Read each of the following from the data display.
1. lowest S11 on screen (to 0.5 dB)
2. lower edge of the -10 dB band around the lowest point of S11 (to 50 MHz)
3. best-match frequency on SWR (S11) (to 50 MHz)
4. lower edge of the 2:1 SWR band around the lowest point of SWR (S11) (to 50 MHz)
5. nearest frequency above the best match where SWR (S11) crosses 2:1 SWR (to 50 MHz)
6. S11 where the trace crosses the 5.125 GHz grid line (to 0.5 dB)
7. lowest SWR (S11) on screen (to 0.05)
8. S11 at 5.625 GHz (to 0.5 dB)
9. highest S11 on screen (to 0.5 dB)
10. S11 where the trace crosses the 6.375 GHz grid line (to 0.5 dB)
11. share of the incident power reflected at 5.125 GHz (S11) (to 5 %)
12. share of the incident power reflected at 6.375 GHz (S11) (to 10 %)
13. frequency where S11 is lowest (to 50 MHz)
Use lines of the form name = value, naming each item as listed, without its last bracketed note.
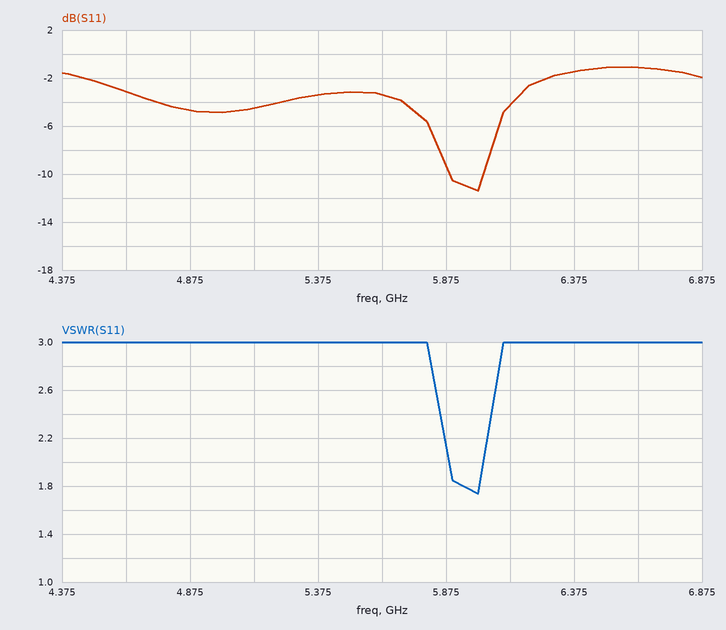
lowest S11 on screen = -11.5 dB
lower edge of the -10 dB band around the lowest point of S11 = 5.90 GHz
best-match frequency on SWR (S11) = 6.00 GHz
lower edge of the 2:1 SWR band around the lowest point of SWR (S11) = 5.90 GHz
nearest frequency above the best match where SWR (S11) crosses 2:1 SWR = 6.00 GHz
S11 where the trace crosses the 5.125 GHz grid line = -4.5 dB
lowest SWR (S11) on screen = 1.75
S11 at 5.625 GHz = -3.5 dB
highest S11 on screen = -1.0 dB
S11 where the trace crosses the 6.375 GHz grid line = -1.5 dB
share of the incident power reflected at 5.125 GHz (S11) = 35 %
share of the incident power reflected at 6.375 GHz (S11) = 70 %
frequency where S11 is lowest = 6.00 GHz
